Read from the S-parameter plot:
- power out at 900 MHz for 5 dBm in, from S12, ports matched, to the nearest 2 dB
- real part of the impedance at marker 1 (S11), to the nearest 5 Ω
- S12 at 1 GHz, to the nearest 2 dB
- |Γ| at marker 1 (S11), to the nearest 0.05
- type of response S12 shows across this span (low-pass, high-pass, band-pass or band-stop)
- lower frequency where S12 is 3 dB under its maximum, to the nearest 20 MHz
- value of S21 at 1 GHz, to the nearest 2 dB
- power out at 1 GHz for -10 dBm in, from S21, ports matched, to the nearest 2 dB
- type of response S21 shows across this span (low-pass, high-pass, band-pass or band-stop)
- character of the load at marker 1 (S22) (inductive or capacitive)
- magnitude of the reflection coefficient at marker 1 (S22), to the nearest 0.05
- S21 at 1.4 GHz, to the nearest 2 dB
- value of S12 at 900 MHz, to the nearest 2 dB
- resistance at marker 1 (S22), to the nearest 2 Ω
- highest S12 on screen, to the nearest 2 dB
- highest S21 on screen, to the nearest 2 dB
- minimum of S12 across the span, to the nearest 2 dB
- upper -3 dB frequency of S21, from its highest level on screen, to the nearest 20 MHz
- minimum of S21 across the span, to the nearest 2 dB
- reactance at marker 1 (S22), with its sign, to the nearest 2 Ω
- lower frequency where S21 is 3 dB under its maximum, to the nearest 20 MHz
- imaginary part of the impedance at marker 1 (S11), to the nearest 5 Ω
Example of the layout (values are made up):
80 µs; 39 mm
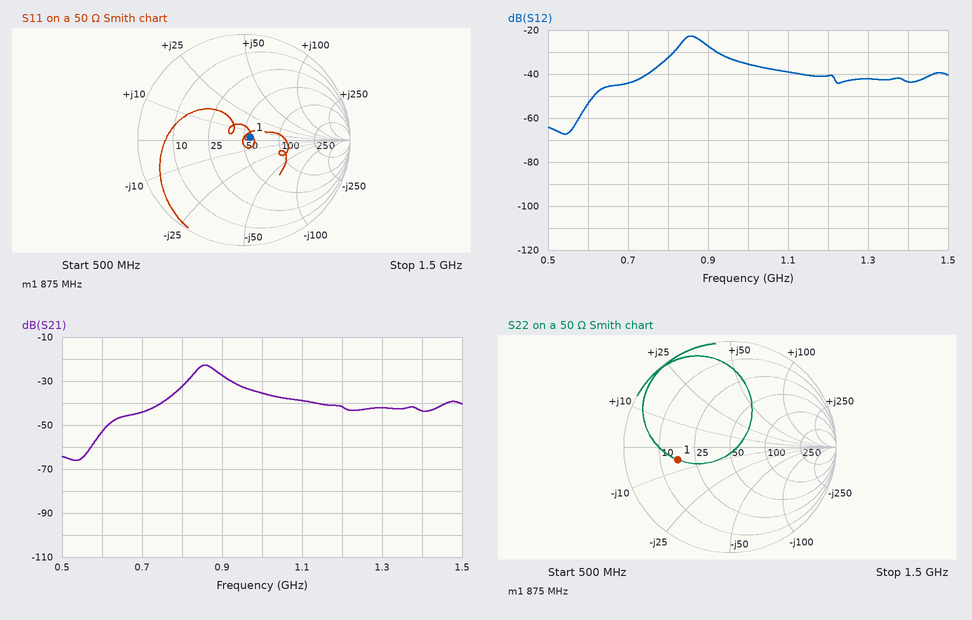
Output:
-22 dBm; 55 Ω; -36 dB; 0.05; band-pass; 840 MHz; -36 dB; -46 dBm; band-pass; capacitive; 0.50; -44 dB; -28 dB; 16 Ω; -22 dB; -22 dB; -68 dB; 880 MHz; -66 dB; -6 Ω; 840 MHz; +5 Ω
